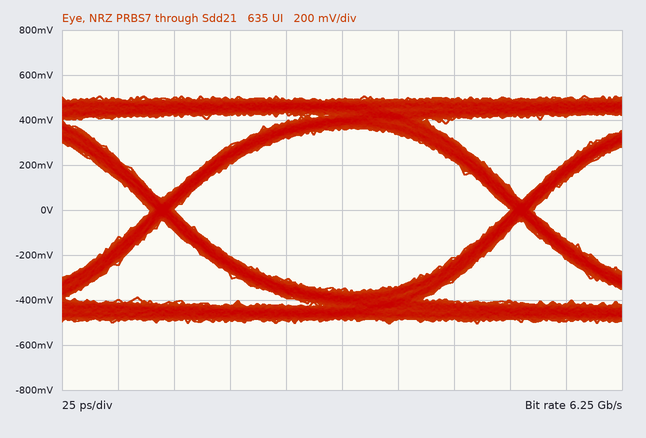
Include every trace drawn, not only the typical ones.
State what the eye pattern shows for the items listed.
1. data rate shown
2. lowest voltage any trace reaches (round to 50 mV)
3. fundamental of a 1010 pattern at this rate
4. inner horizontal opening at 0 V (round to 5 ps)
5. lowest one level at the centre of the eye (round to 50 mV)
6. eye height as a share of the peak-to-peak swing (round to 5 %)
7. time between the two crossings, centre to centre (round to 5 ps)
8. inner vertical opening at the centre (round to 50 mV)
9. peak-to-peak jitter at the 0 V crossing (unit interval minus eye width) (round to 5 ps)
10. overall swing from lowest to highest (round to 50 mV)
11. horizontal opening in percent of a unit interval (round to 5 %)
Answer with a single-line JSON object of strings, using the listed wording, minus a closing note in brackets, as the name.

{"data rate shown": "6.25 Gb/s", "lowest voltage any trace reaches": "-500 mV", "fundamental of a 1010 pattern at this rate": "3.125 GHz", "inner horizontal opening at 0 V": "150 ps", "lowest one level at the centre of the eye": "350 mV", "eye height as a share of the peak-to-peak swing": "70 %", "time between the two crossings, centre to centre": "160 ps", "inner vertical opening at the centre": "700 mV", "peak-to-peak jitter at the 0 V crossing (unit interval minus eye width)": "10 ps", "overall swing from lowest to highest": "1.00 V", "horizontal opening in percent of a unit interval": "95 %"}
